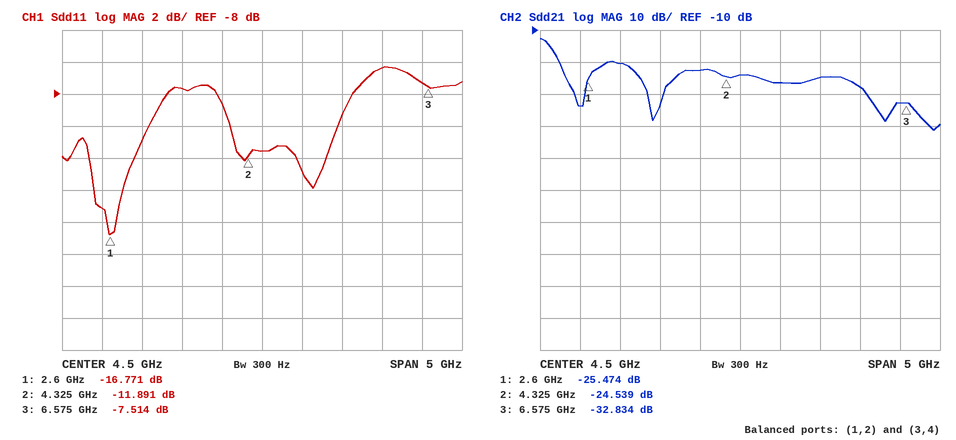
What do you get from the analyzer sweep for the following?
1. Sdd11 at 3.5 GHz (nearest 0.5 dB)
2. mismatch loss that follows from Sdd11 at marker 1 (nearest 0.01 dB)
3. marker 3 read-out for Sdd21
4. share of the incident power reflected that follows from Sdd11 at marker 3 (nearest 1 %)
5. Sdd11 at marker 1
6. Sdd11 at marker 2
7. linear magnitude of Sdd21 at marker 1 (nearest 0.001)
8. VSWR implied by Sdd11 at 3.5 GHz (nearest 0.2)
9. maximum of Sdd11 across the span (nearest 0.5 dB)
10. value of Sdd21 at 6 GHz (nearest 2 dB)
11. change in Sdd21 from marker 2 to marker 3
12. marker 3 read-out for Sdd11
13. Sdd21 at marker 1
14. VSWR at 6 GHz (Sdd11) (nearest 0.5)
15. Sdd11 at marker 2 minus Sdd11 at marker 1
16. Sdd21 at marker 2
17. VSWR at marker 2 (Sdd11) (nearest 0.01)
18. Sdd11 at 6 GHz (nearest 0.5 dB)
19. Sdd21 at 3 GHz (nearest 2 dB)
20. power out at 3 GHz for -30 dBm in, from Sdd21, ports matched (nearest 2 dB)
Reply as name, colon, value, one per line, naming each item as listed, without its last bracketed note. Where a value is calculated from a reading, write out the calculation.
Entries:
Sdd11 at 3.5 GHz: -7.5 dB
mismatch loss that follows from Sdd11 at marker 1: −10 log10(1 − 10^(-16.771/10)) ≈ 0.09 dB
marker 3 read-out for Sdd21: -32.834 dB
share of the incident power reflected that follows from Sdd11 at marker 3: 10^(-7.514/10) ≈ 18 %
Sdd11 at marker 1: -16.771 dB
Sdd11 at marker 2: -11.891 dB
linear magnitude of Sdd21 at marker 1: 10^(-25.474/20) ≈ 0.053
VSWR implied by Sdd11 at 3.5 GHz: |Γ| = 10^(-7.5/20) = 0.4217; VSWR = (1 + 0.4217)/(1 − 0.4217) ≈ 2.46, so 2.4 to the nearest 0.2
maximum of Sdd11 across the span: -6.5 dB
value of Sdd21 at 6 GHz: -28 dB
change in Sdd21 from marker 2 to marker 3: -32.834 − (-24.539) = -8.295 dB
marker 3 read-out for Sdd11: -7.514 dB
Sdd21 at marker 1: -25.474 dB
VSWR at 6 GHz (Sdd11): |Γ| = 10^(-6.5/20) = 0.4732; VSWR = (1 + 0.4732)/(1 − 0.4732) ≈ 2.80, so 3.0 to the nearest 0.5
Sdd11 at marker 2 minus Sdd11 at marker 1: -11.891 − (-16.771) = 4.880 dB
Sdd21 at marker 2: -24.539 dB
VSWR at marker 2 (Sdd11): (1 + 0.2544)/(1 − 0.2544) ≈ 1.68
Sdd11 at 6 GHz: -6.5 dB
Sdd21 at 3 GHz: -20 dB
power out at 3 GHz for -30 dBm in, from Sdd21, ports matched: -30 dBm + (-20 dB) = -50 dBm
